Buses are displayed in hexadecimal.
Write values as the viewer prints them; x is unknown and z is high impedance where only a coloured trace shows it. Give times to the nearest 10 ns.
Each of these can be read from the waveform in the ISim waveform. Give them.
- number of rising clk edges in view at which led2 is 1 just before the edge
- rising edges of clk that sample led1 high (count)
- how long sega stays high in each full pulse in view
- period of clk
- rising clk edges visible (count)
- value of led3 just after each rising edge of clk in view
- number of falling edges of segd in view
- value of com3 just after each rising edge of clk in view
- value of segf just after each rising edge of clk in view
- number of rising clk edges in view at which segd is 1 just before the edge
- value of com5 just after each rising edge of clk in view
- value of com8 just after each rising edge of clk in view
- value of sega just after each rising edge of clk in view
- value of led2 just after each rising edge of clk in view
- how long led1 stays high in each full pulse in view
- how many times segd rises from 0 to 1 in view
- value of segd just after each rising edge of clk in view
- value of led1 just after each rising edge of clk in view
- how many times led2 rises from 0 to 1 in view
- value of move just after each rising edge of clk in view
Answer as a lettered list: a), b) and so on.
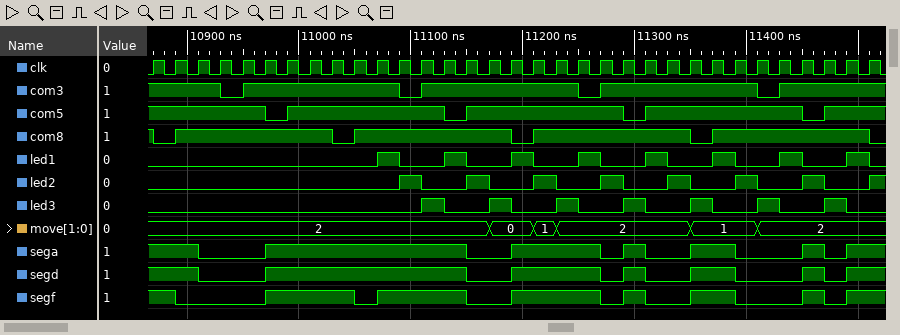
a) 7
b) 8
c) 180 ns, 80 ns, 20 ns, 40 ns, 20 ns
d) 20 ns
e) 33
f) 0 0 0 0 0 0 0 0 0 0 0 0 1 0 0 1 0 0 1 0 0 1 0 0 1 0 0 1 0 0 1 0 0
g) 6
h) 1 1 1 0 1 1 1 1 1 1 1 0 1 1 1 1 1 1 1 0 1 1 1 1 1 1 1 0 1 1 1 1 1
i) 1 0 0 0 0 1 1 1 1 0 1 1 1 1 0 0 1 1 1 1 0 1 0 0 1 1 0 0 0 1 0 1 1
j) 21
k) 1 1 1 1 1 0 1 1 1 1 1 1 1 0 1 1 1 1 1 1 1 0 1 1 1 1 1 1 1 0 1 1 1
l) 0 1 1 1 1 1 1 1 0 1 1 1 1 1 1 1 0 1 1 1 1 1 1 1 0 1 1 1 1 1 1 1 0
m) 1 1 0 0 0 1 1 1 1 1 1 1 1 1 0 0 1 1 1 1 0 1 0 0 1 1 0 0 0 1 0 1 1
n) 0 0 0 0 0 0 0 0 0 0 0 1 0 0 1 0 0 1 0 0 1 0 0 1 0 0 1 0 0 1 0 0 1
o) 20 ns, 20 ns, 20 ns, 20 ns, 20 ns, 20 ns, 20 ns, 20 ns
p) 6
q) 1 1 0 0 0 1 1 1 1 1 1 1 1 1 0 0 1 1 1 1 0 1 0 0 1 1 0 0 0 1 0 1 1
r) 0 0 0 0 0 0 0 0 0 0 1 0 0 1 0 0 1 0 0 1 0 0 1 0 0 1 0 0 1 0 0 1 0
s) 8
t) 2, 2, 2, 2, 2, 2, 2, 2, 2, 2, 2, 2, 2, 2, 2, 0, 0, 1, 2, 2, 2, 2, 2, 2, 1, 1, 1, 2, 2, 2, 2, 2, 2
